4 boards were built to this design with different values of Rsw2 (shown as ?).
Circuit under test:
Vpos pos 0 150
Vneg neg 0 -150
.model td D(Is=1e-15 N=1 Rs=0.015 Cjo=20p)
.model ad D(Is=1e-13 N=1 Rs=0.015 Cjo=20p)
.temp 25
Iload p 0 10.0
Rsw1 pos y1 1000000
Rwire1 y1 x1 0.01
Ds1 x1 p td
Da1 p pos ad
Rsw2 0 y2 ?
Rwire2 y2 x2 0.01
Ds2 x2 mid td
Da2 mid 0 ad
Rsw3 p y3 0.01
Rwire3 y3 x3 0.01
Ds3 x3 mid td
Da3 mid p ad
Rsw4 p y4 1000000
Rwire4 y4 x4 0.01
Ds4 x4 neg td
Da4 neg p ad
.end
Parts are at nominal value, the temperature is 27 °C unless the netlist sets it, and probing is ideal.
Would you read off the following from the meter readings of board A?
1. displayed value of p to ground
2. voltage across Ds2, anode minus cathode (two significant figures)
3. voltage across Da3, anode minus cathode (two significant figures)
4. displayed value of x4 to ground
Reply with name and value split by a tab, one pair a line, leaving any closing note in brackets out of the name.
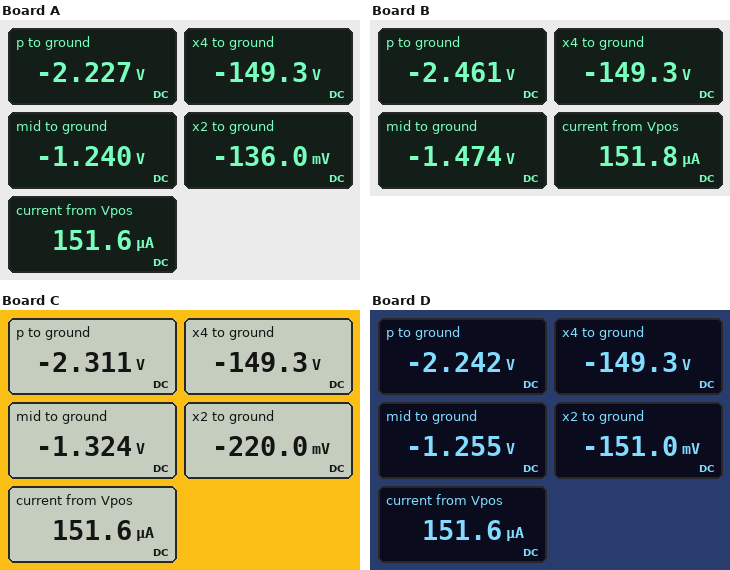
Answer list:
displayed value of p to ground	-2.227 V
voltage across Ds2, anode minus cathode	1.1 V
voltage across Da3, anode minus cathode	990 mV
displayed value of x4 to ground	-149.3 V
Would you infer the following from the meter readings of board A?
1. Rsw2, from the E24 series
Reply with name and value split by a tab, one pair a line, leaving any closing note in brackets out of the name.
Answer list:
Rsw2, from the E24 series	3.6 mΩ
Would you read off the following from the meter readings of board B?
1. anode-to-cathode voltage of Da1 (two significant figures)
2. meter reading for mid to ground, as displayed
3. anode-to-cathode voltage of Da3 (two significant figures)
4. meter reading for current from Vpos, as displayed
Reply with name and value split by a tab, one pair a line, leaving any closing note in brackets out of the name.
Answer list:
anode-to-cathode voltage of Da1	-150 V
meter reading for mid to ground, as displayed	-1.474 V
anode-to-cathode voltage of Da3	990 mV
meter reading for current from Vpos, as displayed	151.8 µA
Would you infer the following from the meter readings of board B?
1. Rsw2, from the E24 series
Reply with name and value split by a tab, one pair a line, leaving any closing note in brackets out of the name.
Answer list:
Rsw2, from the E24 series	0.027 Ω
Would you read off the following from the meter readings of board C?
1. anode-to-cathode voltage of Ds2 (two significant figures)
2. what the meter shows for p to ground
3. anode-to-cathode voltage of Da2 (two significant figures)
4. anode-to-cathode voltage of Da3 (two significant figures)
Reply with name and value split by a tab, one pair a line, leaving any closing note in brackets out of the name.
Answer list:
anode-to-cathode voltage of Ds2	1.1 V
what the meter shows for p to ground	-2.311 V
anode-to-cathode voltage of Da2	-1.3 V
anode-to-cathode voltage of Da3	990 mV
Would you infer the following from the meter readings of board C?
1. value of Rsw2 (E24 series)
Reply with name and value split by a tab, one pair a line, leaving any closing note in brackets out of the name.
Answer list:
value of Rsw2	0.012 Ω
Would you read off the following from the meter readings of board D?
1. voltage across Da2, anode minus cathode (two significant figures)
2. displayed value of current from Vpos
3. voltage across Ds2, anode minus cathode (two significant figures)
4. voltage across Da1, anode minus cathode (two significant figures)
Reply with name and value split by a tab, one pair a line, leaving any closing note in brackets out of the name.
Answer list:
voltage across Da2, anode minus cathode	-1.3 V
displayed value of current from Vpos	151.6 µA
voltage across Ds2, anode minus cathode	1.1 V
voltage across Da1, anode minus cathode	-150 V
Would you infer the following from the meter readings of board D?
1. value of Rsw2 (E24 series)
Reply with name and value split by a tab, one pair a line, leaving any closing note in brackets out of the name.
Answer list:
value of Rsw2	5.1 mΩ
